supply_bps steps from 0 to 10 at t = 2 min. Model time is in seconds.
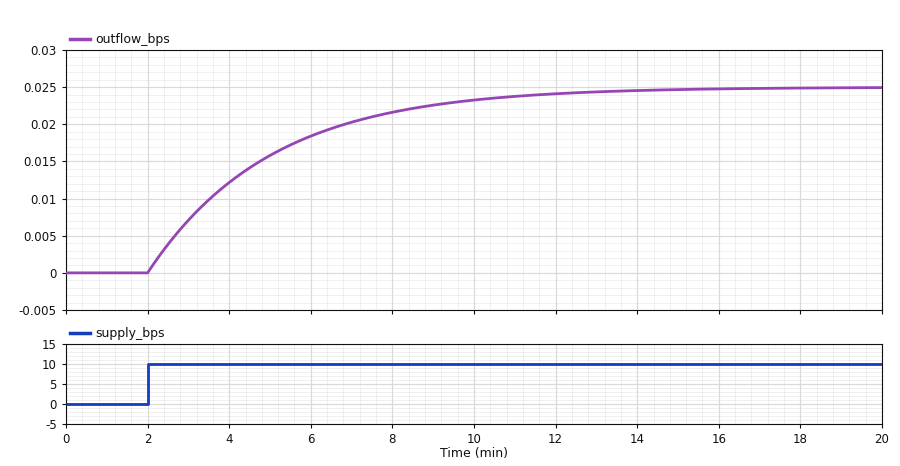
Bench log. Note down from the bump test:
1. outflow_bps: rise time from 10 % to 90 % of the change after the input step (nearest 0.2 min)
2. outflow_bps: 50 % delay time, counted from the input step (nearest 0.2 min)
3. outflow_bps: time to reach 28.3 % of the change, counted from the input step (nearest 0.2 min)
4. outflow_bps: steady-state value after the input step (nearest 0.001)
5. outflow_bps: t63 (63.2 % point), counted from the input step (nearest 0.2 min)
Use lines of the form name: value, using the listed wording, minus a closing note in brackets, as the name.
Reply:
outflow_bps: rise time from 10 % to 90 % of the change after the input step: 6.6 min
outflow_bps: 50 % delay time, counted from the input step: 2.0 min
outflow_bps: time to reach 28.3 % of the change, counted from the input step: 1.0 min
outflow_bps: steady-state value after the input step: 0.025
outflow_bps: t63 (63.2 % point), counted from the input step: 3.0 min
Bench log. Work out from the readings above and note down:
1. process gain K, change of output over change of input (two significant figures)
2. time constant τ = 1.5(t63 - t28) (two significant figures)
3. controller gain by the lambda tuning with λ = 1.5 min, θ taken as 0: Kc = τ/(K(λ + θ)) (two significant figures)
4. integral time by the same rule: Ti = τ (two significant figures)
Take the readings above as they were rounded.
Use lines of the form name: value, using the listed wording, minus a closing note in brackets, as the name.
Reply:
process gain K, change of output over change of input: 0.0025
time constant τ = 1.5(t63 - t28): 3.0 min
controller gain by the lambda tuning with λ = 1.5 min, θ taken as 0: Kc = τ/(K(λ + θ)): 800
integral time by the same rule: Ti = τ: 3.0 min
